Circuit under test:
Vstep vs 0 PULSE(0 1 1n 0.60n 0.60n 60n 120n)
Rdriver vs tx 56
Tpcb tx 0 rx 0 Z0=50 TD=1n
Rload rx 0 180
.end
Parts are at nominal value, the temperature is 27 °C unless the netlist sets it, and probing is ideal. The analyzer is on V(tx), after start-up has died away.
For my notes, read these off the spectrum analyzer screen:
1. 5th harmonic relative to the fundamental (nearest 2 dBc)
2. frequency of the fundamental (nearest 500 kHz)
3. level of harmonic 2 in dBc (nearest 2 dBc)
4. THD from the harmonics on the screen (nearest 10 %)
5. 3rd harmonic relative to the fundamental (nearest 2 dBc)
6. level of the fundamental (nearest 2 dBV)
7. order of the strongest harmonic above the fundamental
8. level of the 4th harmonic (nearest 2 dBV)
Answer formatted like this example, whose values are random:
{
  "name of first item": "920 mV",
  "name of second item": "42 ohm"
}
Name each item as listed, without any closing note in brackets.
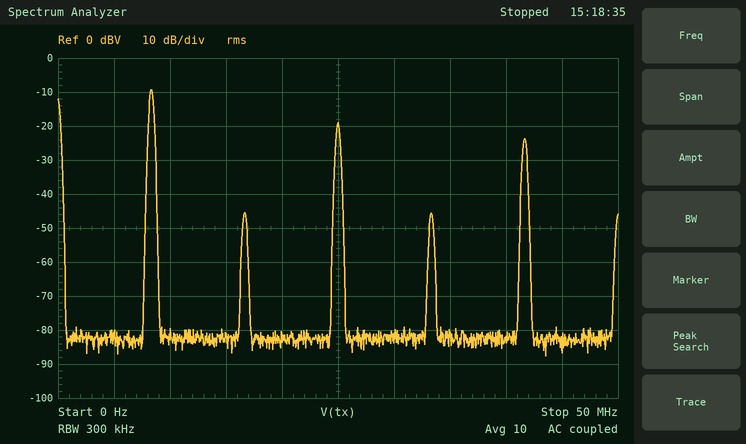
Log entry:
{
  "5th harmonic relative to the fundamental": "-14 dBc",
  "frequency of the fundamental": "8.5 MHz",
  "level of harmonic 2 in dBc": "-36 dBc",
  "THD from the harmonics on the screen": "40 %",
  "3rd harmonic relative to the fundamental": "-10 dBc",
  "level of the fundamental": "-10 dBV",
  "order of the strongest harmonic above the fundamental": "3",
  "level of the 4th harmonic": "-46 dBV"
}
